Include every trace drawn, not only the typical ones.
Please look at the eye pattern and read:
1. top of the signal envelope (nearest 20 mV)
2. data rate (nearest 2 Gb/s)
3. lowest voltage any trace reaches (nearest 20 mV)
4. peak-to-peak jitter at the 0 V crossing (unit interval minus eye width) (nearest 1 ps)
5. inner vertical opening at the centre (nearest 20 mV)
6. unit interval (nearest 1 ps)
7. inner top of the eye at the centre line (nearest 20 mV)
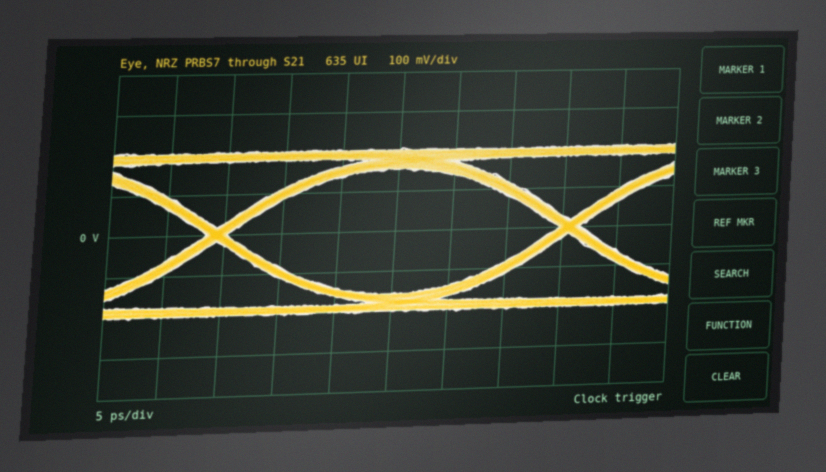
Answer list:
200 mV
32 Gb/s
-200 mV
2 ps
320 mV
31 ps
160 mV
